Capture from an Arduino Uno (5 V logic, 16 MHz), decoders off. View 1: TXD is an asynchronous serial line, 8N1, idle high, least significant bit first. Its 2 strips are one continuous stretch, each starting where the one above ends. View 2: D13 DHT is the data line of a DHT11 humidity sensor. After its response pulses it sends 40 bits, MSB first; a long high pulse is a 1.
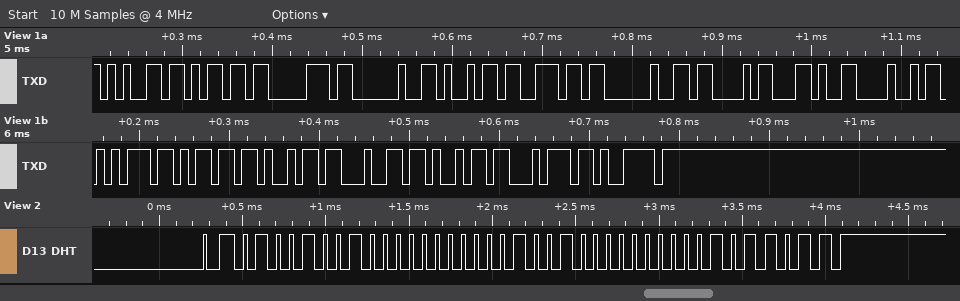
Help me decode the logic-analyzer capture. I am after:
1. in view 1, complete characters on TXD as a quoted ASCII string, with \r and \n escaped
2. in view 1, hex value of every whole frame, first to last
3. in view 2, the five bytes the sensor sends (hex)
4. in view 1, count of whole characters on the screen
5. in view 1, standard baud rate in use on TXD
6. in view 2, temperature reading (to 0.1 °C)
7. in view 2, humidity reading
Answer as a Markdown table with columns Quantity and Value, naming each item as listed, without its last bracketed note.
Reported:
| Quantity | Value |
|---|---|
| in view 1, complete characters on TXD as a quoted ASCII string, with \r and \n escaped | "emp in C,Humidity" |
| in view 1, hex value of every whole frame, first to last | 0x65 0x6D 0x70 0x20 0x69 0x6E 0x20 0x43 0x2C 0x48 0x75 0x6D 0x69 0x64 0x69 0x74 0x79 |
| in view 2, the five bytes the sensor sends | 49 00 12 00 5B |
| in view 1, count of whole characters on the screen | 17 |
| in view 1, standard baud rate in use on TXD | 115200 baud |
| in view 2, temperature reading | 18.0 °C |
| in view 2, humidity reading | 73 % |
